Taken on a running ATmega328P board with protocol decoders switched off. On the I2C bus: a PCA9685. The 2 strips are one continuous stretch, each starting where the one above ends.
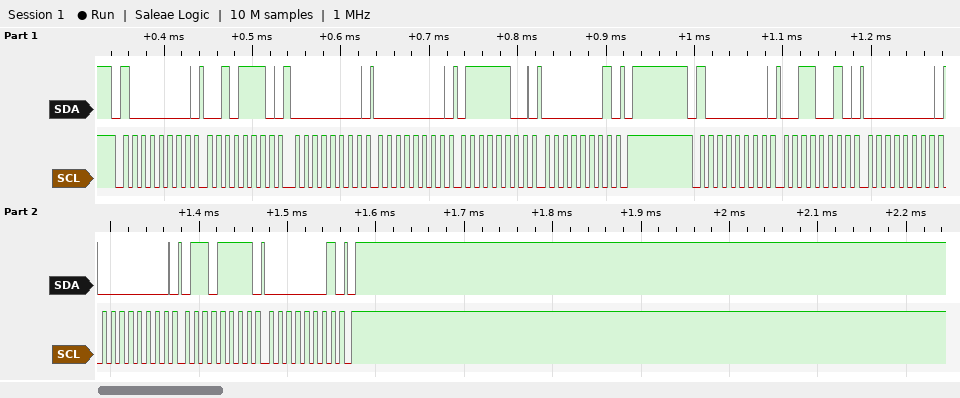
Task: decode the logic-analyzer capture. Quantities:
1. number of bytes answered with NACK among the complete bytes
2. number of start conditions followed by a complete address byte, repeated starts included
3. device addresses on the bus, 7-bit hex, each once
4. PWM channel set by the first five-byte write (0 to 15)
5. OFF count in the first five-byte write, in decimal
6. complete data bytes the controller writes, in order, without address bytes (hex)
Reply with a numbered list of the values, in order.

1. 0
2. 2
3. 0x40
4. 10
5. 380
6. 2E 00 00 7C 01 32 00 00 6F 01
